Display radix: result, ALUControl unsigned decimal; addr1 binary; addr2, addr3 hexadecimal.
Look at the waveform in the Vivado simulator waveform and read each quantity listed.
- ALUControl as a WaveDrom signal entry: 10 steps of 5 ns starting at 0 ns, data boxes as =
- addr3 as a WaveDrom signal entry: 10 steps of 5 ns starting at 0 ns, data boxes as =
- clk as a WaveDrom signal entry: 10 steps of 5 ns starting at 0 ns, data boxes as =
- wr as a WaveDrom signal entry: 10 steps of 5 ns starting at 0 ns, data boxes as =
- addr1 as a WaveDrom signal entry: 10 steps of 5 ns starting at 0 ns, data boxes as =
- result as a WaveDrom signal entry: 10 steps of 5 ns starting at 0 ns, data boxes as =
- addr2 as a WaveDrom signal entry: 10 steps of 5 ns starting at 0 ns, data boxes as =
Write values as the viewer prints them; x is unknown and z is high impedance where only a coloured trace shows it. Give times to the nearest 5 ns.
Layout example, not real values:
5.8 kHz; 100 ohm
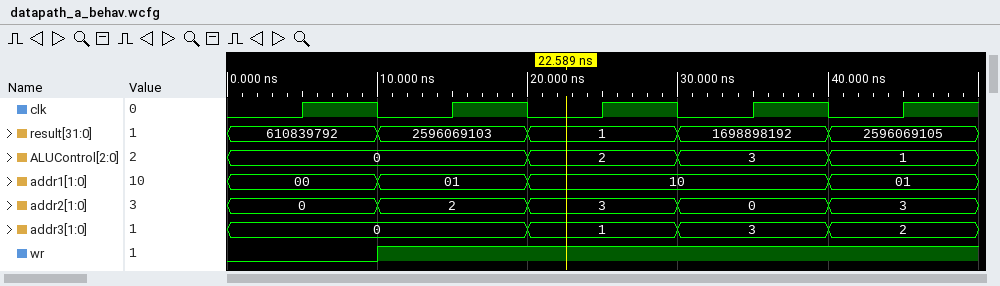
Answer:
{name: 'ALUControl', wave: '=...=.=.=.', data: '0 2 3 1'}; {name: 'addr3', wave: '=...=.=.=.', data: '0 1 3 2'}; {name: 'clk', wave: '0101010101'}; {name: 'wr', wave: '0.1.......'}; {name: 'addr1', wave: '=.=.=...=.', data: '00 01 10 01'}; {name: 'result', wave: '=.=.=.=.=.', data: '610839792 2596069103 1 1698898192 2596069105'}; {name: 'addr2', wave: '=.=.=.=.=.', data: '0 2 3 0 3'}
